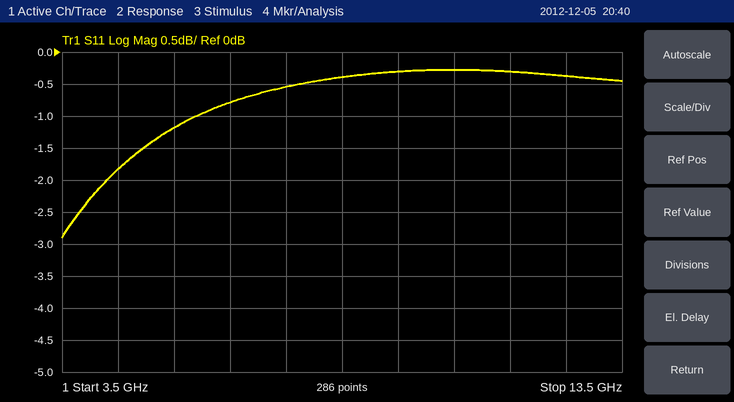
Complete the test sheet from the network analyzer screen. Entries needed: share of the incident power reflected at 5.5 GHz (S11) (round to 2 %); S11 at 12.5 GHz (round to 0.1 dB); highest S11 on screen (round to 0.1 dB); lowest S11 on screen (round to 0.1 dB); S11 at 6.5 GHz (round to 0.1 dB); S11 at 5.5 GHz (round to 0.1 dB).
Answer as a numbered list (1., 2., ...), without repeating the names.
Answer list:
1. 76 %
2. -0.4 dB
3. -0.3 dB
4. -2.9 dB
5. -0.8 dB
6. -1.2 dB
